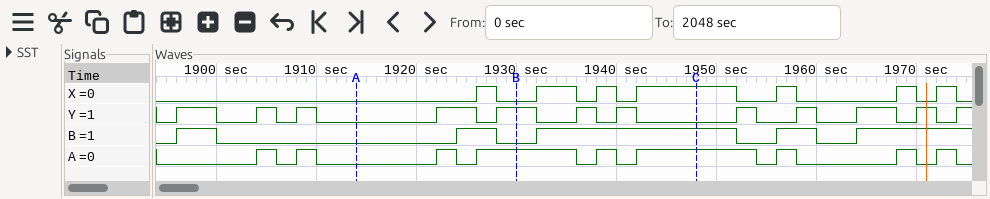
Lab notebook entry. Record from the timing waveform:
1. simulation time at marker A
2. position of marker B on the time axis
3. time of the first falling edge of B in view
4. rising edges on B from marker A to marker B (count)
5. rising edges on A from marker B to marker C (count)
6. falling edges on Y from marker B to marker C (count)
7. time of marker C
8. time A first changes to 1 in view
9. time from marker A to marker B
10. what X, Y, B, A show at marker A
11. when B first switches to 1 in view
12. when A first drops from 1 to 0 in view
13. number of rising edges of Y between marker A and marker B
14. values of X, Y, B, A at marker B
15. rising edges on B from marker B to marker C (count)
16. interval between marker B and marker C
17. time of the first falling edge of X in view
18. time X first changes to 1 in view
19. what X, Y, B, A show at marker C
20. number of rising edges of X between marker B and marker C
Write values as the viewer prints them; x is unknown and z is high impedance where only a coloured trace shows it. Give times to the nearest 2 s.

1914 s
1930 s
1900 s
1
2
3
1948 s
1904 s
16 s
X=0, Y=0, B=0, A=0
1896 s
1906 s
2
X=0, Y=1, B=0, A=1
1
18 s
1928 s
1926 s
X=1, Y=0, B=1, A=1
3
